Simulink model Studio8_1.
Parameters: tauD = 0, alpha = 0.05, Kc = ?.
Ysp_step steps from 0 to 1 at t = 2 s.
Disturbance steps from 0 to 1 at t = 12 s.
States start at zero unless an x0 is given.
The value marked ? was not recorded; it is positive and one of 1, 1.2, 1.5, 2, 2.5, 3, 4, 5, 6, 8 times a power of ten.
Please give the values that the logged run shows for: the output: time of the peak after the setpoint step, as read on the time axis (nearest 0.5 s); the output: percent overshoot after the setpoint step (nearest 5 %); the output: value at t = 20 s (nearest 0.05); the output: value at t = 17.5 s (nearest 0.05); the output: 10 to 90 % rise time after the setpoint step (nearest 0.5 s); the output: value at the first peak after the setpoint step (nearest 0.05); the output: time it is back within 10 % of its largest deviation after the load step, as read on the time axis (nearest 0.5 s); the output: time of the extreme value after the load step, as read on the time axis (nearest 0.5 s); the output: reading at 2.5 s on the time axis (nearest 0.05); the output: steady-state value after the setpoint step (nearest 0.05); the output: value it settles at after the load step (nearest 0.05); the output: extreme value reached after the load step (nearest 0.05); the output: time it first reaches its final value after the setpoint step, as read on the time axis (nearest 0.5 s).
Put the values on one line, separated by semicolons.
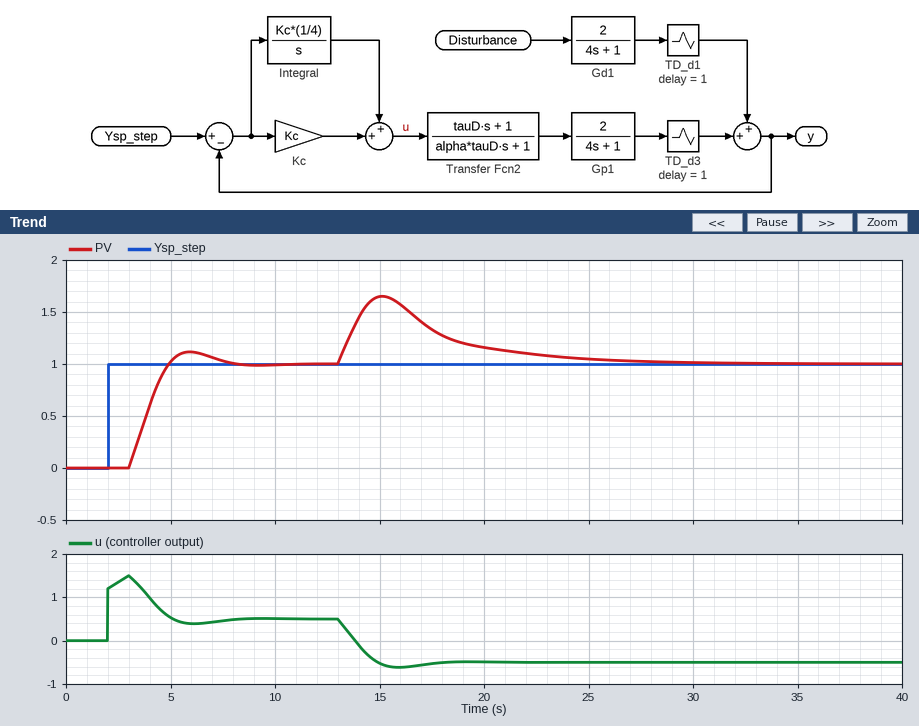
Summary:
6.0 s; 10 %; 1.15; 1.35; 1.5 s; 1.10; 24.0 s; 15.0 s; 0.00; 1.00; 1.00; 1.65; 5.0 s
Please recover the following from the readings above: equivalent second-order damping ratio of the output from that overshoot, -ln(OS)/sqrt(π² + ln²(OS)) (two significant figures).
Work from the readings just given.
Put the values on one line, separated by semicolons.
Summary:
0.59
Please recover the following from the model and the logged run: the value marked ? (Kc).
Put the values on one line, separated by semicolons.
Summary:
1.2
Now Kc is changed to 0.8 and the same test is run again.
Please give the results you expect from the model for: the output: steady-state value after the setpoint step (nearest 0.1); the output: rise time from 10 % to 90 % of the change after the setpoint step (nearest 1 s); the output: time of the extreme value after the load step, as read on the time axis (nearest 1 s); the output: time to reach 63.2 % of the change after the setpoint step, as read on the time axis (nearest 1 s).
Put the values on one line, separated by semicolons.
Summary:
1.0; 3 s; 16 s; 5 s
